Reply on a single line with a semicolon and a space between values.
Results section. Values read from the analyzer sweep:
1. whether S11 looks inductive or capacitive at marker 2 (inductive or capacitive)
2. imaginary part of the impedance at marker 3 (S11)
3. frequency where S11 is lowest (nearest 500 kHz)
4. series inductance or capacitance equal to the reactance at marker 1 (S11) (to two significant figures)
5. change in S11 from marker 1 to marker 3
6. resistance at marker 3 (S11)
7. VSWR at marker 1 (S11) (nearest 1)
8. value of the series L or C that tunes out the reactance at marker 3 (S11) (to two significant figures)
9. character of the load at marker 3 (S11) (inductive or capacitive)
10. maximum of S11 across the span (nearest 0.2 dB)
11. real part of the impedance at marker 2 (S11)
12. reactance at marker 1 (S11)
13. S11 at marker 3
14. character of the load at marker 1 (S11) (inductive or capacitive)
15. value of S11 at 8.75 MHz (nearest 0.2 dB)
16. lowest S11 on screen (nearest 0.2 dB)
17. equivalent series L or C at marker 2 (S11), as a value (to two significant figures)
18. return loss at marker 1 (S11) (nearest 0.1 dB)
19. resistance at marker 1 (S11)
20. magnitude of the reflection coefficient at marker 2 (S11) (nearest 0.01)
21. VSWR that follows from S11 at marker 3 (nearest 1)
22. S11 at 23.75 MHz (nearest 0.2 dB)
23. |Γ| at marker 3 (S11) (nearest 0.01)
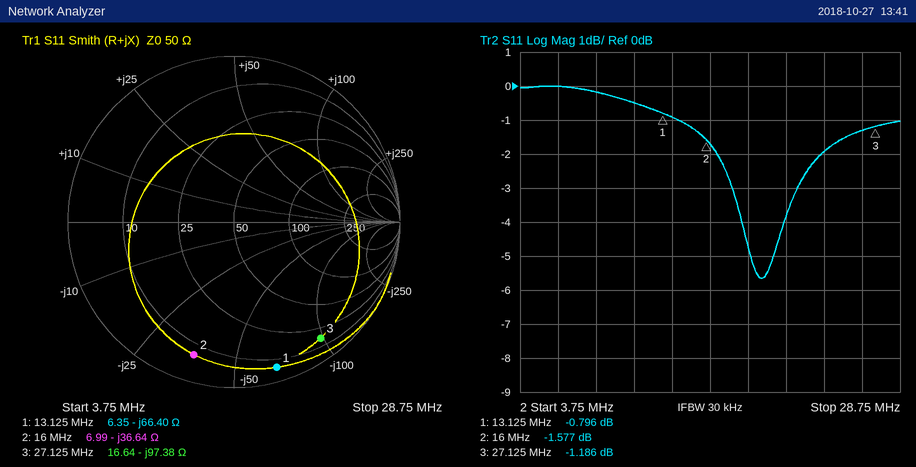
capacitive; -97.38 Ω; 19.5 MHz; 180 pF; -0.390 dB; 16.64 Ω; 22; 570 nH; capacitive; 0.0 dB; 6.99 Ω; -66.40 Ω; -1.186 dB; capacitive; -0.2 dB; -5.6 dB; 270 pF; 0.8 dB; 6.35 Ω; 0.83; 15; -2.0 dB; 0.87
